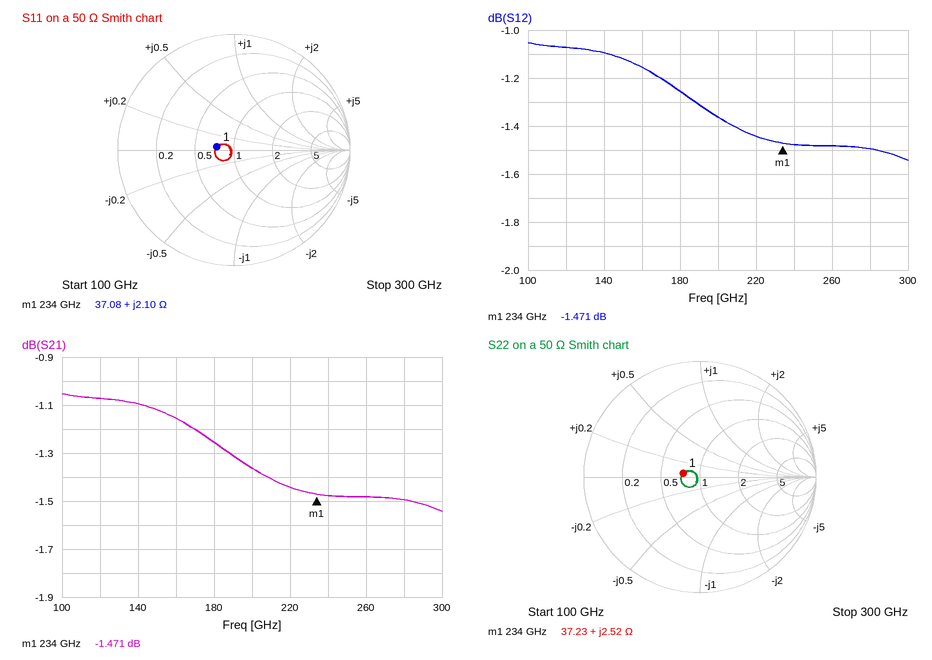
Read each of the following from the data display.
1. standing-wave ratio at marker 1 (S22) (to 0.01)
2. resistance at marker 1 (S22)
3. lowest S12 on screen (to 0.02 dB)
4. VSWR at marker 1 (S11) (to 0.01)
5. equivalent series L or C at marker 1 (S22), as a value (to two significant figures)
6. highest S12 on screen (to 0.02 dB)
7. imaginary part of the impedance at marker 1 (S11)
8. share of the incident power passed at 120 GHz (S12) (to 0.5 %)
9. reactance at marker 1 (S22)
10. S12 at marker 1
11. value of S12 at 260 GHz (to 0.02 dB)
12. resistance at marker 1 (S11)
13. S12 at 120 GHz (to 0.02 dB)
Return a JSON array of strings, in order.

["1.35", "37.23 Ω", "-1.54 dB", "1.35", "1.7 pH", "-1.06 dB", "+2.10 Ω", "78.0 %", "+2.52 Ω", "-1.471 dB", "-1.48 dB", "37.08 Ω", "-1.08 dB"]
